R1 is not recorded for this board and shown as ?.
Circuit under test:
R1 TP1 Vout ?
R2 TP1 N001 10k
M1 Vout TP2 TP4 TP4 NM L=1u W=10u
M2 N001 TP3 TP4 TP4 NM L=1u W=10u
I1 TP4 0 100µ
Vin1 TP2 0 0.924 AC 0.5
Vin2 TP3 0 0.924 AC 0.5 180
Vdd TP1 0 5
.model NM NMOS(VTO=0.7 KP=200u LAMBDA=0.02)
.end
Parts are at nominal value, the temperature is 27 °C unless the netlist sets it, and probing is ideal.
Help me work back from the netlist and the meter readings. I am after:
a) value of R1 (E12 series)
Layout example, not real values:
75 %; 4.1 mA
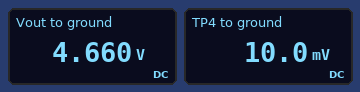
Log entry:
6.8 kΩ
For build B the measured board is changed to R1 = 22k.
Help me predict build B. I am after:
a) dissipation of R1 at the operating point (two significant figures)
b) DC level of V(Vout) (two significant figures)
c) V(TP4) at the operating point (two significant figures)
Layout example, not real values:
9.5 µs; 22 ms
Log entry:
54 µW; 3.9 V; 9.2 mV
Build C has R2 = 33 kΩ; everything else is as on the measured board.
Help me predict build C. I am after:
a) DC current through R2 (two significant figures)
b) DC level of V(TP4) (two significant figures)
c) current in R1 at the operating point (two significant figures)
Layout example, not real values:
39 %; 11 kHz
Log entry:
49 µA; 8.8 mV; 51 µA
